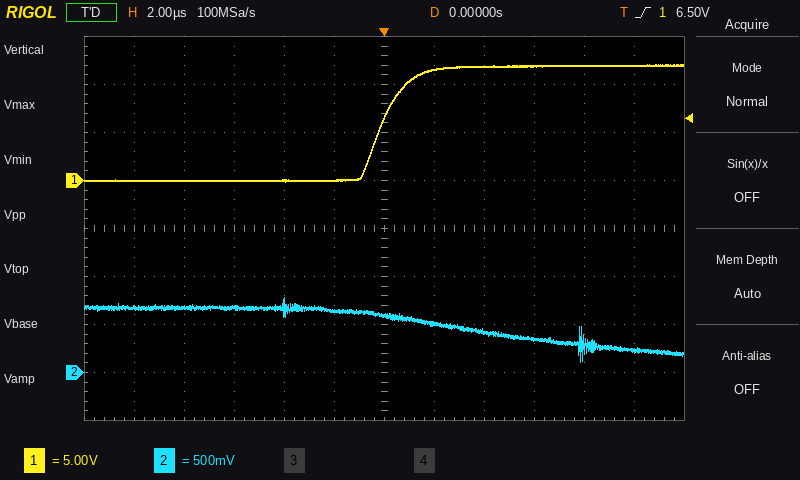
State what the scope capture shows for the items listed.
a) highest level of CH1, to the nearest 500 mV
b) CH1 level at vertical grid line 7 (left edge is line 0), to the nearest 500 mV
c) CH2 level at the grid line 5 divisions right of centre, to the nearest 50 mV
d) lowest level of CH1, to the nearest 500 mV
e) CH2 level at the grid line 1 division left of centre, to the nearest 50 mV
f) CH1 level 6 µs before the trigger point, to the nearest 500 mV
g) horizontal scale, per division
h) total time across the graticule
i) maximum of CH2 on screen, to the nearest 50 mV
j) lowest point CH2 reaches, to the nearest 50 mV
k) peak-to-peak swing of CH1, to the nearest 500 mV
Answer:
12.0 V
11.5 V
250 mV
0.0 V
650 mV
0.0 V
2 µs
24 µs
800 mV
100 mV
12.0 V
